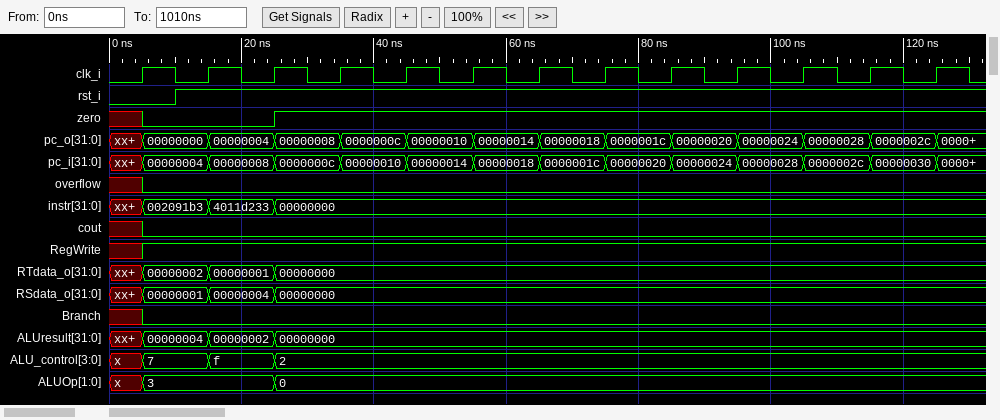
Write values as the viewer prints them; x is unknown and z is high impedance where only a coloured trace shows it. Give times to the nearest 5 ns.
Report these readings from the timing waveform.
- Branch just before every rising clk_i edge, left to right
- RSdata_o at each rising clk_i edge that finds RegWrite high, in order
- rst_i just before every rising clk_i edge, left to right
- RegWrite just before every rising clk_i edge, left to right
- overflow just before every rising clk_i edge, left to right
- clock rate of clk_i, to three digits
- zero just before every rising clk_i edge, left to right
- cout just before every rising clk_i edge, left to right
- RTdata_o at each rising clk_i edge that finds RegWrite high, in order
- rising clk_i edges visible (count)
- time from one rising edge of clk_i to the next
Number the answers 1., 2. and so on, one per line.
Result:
1. x 0 0 0 0 0 0 0 0 0 0 0 0
2. 00000001, 00000004, 00000000, 00000000, 00000000, 00000000, 00000000, 00000000, 00000000, 00000000, 00000000, 00000000
3. 0 1 1 1 1 1 1 1 1 1 1 1 1
4. x 1 1 1 1 1 1 1 1 1 1 1 1
5. x 0 0 0 0 0 0 0 0 0 0 0 0
6. 100 MHz
7. x 0 0 1 1 1 1 1 1 1 1 1 1
8. x 0 0 0 0 0 0 0 0 0 0 0 0
9. 00000002, 00000001, 00000000, 00000000, 00000000, 00000000, 00000000, 00000000, 00000000, 00000000, 00000000, 00000000
10. 13
11. 10 ns
